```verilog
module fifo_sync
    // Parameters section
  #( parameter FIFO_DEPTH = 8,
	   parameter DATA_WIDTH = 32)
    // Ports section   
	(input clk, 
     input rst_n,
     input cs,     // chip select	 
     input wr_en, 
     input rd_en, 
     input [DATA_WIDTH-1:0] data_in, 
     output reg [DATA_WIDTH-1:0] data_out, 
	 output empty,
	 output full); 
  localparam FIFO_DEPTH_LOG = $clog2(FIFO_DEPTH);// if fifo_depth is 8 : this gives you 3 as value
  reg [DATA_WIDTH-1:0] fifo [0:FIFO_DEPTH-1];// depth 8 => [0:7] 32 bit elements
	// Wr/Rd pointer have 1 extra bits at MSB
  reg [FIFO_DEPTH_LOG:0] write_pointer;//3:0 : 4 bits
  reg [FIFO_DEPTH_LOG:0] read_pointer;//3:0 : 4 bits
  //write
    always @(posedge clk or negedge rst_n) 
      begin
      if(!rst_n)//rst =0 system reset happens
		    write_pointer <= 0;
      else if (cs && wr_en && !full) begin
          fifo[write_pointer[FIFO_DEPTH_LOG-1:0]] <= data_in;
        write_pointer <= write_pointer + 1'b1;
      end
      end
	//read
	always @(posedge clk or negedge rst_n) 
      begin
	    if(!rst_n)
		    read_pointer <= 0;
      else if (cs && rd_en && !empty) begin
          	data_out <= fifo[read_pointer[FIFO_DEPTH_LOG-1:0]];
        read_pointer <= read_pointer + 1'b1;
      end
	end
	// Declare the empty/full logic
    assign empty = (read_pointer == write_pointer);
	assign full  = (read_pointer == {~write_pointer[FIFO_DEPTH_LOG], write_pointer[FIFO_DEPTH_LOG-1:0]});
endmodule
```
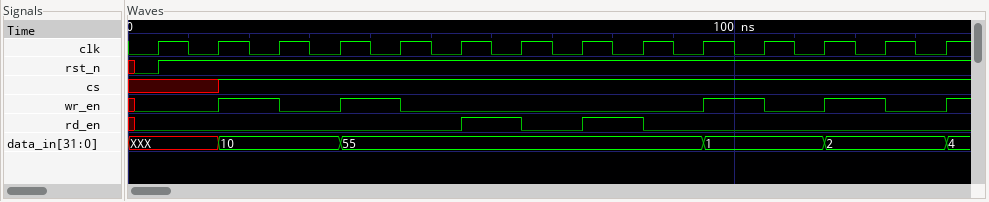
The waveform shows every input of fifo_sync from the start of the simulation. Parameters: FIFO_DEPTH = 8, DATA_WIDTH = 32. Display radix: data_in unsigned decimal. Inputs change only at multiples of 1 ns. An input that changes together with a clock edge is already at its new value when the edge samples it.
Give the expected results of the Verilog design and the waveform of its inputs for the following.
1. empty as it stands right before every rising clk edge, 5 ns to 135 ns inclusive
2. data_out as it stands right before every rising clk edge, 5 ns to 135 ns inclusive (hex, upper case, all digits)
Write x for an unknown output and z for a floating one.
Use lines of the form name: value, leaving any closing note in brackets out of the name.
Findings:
empty as it stands right before every rising clk edge, 5 ns to 135 ns inclusive: 1 1 0 0 0 0 0 0 1 1 0 0 0 0
data_out as it stands right before every rising clk edge, 5 ns to 135 ns inclusive: x, x, x, x, x, x, 0000000A, 0000000A, 00000037, 00000037, 00000037, 00000037, 00000037, 00000037
